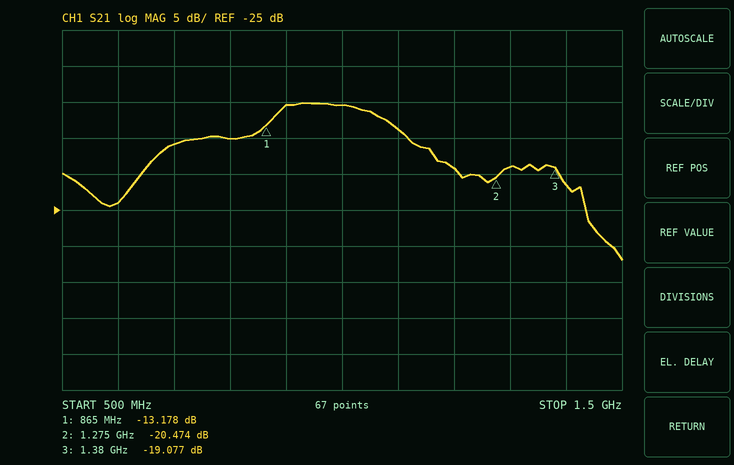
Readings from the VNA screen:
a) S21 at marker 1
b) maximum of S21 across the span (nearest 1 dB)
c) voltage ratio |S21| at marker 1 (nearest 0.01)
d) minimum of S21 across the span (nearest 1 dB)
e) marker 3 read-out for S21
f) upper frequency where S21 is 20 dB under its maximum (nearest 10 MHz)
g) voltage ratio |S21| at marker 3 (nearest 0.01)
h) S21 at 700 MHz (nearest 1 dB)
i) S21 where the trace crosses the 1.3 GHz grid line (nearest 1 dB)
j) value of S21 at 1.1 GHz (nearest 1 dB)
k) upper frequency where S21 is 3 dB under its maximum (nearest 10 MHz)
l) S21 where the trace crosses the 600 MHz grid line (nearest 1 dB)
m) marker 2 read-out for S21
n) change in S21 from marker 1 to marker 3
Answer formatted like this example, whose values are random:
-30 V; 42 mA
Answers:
-13.178 dB; -10 dB; 0.22; -32 dB; -19.077 dB; 1.48 GHz; 0.11; -16 dB; -19 dB; -14 dB; 1.09 GHz; -24 dB; -20.474 dB; -5.899 dB
